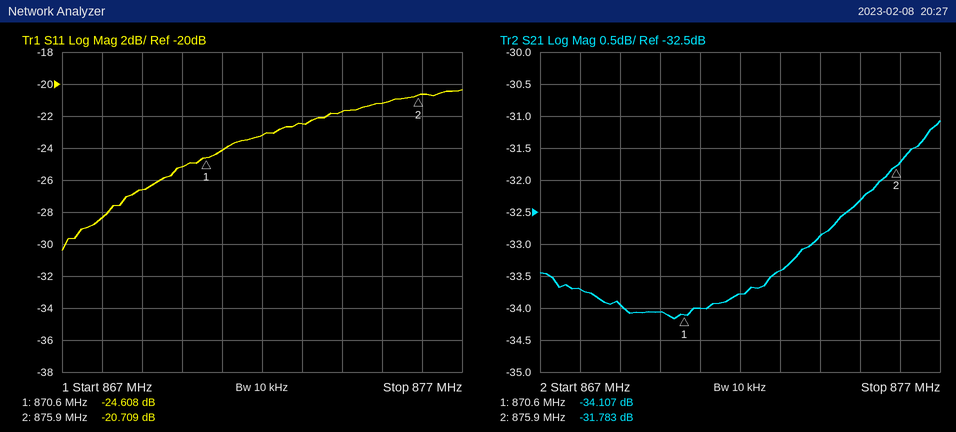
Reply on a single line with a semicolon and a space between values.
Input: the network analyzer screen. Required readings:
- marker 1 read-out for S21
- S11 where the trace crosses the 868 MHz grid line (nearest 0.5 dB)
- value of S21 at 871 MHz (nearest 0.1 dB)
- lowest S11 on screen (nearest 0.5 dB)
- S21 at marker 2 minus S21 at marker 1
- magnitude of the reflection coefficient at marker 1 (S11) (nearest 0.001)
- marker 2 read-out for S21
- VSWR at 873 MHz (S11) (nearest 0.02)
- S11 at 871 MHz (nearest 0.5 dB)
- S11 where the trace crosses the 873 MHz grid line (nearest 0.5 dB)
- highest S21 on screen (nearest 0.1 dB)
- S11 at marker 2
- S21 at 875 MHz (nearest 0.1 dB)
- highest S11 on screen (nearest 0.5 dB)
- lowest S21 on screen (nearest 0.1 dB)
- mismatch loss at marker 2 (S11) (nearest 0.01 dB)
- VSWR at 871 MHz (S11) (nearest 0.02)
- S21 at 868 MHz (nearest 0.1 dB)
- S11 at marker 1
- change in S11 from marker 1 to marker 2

-34.107 dB; -28.5 dB; -34.0 dB; -30.5 dB; 2.324 dB; 0.059; -31.783 dB; 1.16; -24.0 dB; -22.5 dB; -31.1 dB; -20.709 dB; -32.3 dB; -20.5 dB; -34.2 dB; 0.04 dB; 1.14; -33.7 dB; -24.608 dB; 3.899 dB
